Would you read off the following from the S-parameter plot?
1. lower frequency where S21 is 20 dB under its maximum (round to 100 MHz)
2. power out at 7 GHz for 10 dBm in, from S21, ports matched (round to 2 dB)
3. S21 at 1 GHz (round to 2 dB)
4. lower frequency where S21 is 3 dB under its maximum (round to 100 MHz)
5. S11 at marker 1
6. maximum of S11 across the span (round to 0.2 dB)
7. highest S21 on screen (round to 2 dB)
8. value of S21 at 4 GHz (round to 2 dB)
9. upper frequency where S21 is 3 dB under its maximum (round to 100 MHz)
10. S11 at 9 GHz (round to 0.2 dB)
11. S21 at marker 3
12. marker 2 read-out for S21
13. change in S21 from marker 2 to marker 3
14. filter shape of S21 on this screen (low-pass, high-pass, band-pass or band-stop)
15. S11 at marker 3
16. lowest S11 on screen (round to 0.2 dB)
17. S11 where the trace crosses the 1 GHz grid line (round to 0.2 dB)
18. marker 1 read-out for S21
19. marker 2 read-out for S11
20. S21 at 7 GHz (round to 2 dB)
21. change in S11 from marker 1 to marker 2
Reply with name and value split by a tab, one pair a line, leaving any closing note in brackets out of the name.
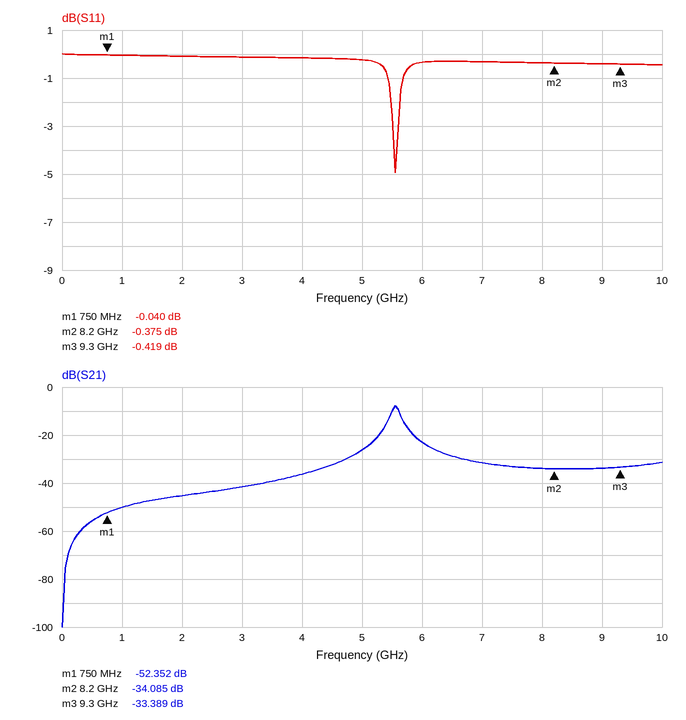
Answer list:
lower frequency where S21 is 20 dB under its maximum	4.9 GHz
power out at 7 GHz for 10 dBm in, from S21, ports matched	-22 dBm
S21 at 1 GHz	-50 dB
lower frequency where S21 is 3 dB under its maximum	5.5 GHz
S11 at marker 1	-0.040 dB
maximum of S11 across the span	0.0 dB
highest S21 on screen	-8 dB
value of S21 at 4 GHz	-36 dB
upper frequency where S21 is 3 dB under its maximum	5.6 GHz
S11 at 9 GHz	-0.4 dB
S21 at marker 3	-33.389 dB
marker 2 read-out for S21	-34.085 dB
change in S21 from marker 2 to marker 3	0.696 dB
filter shape of S21 on this screen	band-pass
S11 at marker 3	-0.419 dB
lowest S11 on screen	-5.0 dB
S11 where the trace crosses the 1 GHz grid line	0.0 dB
marker 1 read-out for S21	-52.352 dB
marker 2 read-out for S11	-0.375 dB
S21 at 7 GHz	-32 dB
change in S11 from marker 1 to marker 2	-0.335 dB
